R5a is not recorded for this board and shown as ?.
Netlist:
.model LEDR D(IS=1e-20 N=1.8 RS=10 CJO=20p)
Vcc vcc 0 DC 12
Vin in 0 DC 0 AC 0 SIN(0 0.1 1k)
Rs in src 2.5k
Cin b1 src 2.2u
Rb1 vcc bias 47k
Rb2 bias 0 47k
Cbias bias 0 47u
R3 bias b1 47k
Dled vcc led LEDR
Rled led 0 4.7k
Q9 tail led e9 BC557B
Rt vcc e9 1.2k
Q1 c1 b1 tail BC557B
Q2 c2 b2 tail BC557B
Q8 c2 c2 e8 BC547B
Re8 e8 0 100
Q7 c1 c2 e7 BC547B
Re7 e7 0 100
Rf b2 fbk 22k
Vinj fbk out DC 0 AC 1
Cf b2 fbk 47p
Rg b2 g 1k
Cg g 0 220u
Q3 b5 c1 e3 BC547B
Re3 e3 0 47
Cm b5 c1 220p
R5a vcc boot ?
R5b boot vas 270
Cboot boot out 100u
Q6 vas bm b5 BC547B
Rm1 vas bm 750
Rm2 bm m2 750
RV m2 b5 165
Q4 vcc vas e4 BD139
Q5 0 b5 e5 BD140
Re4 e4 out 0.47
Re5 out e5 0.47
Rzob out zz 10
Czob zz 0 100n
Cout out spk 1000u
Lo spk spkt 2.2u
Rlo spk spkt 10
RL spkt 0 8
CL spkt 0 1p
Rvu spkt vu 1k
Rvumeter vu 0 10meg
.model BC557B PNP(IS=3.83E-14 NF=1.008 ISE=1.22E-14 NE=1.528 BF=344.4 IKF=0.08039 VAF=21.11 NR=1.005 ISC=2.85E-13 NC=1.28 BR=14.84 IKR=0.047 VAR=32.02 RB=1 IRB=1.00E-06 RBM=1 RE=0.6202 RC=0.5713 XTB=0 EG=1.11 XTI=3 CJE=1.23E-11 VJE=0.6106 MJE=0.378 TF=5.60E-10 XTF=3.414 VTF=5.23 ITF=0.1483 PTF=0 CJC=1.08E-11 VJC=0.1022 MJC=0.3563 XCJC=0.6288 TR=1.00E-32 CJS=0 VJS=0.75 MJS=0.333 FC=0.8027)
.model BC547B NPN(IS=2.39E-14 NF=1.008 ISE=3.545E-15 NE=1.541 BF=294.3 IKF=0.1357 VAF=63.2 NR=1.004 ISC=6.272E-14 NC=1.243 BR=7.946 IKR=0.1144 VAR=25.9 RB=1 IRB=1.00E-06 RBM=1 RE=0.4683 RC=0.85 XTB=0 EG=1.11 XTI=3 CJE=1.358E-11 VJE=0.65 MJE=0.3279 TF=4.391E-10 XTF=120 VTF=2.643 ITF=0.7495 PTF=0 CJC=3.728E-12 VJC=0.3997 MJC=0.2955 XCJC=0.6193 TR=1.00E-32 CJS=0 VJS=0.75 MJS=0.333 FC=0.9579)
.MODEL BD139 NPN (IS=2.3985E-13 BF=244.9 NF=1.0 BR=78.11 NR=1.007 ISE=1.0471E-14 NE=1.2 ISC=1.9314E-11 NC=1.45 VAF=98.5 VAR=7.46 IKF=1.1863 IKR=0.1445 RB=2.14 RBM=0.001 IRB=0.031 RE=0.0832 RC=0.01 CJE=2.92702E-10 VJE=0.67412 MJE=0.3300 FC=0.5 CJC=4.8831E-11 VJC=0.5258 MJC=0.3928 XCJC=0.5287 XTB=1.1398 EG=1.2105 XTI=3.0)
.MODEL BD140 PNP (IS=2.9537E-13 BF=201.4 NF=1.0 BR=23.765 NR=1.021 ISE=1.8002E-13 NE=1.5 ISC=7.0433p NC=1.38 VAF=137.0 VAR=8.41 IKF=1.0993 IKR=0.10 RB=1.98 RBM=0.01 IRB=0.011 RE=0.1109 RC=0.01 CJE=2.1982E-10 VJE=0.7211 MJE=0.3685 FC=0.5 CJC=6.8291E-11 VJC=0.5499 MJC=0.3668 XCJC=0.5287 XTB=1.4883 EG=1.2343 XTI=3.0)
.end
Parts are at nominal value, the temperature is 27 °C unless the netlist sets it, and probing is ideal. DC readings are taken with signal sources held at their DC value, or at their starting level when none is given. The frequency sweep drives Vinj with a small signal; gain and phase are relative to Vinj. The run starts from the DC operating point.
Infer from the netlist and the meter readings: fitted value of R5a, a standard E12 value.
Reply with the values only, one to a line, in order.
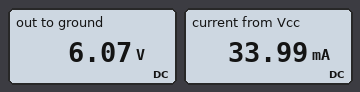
180 Ω
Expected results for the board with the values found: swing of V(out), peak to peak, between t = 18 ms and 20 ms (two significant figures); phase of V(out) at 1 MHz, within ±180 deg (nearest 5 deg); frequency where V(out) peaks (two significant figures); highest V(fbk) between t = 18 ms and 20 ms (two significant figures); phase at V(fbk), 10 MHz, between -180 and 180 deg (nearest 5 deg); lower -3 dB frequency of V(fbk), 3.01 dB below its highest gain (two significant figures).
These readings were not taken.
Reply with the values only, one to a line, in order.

4.3 V
165 deg
4.7 MHz
8.2 V
-5 deg
4.2 MHz
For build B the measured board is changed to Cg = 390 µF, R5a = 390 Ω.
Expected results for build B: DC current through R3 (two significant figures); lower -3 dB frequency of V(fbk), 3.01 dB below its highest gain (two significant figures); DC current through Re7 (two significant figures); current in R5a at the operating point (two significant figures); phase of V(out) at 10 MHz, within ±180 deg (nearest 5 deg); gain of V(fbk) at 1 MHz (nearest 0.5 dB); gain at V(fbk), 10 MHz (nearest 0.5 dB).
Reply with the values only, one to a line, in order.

1.3 µA
3.9 MHz
510 µA
8.0 mA
-25 deg
-9.5 dB
2.0 dB
